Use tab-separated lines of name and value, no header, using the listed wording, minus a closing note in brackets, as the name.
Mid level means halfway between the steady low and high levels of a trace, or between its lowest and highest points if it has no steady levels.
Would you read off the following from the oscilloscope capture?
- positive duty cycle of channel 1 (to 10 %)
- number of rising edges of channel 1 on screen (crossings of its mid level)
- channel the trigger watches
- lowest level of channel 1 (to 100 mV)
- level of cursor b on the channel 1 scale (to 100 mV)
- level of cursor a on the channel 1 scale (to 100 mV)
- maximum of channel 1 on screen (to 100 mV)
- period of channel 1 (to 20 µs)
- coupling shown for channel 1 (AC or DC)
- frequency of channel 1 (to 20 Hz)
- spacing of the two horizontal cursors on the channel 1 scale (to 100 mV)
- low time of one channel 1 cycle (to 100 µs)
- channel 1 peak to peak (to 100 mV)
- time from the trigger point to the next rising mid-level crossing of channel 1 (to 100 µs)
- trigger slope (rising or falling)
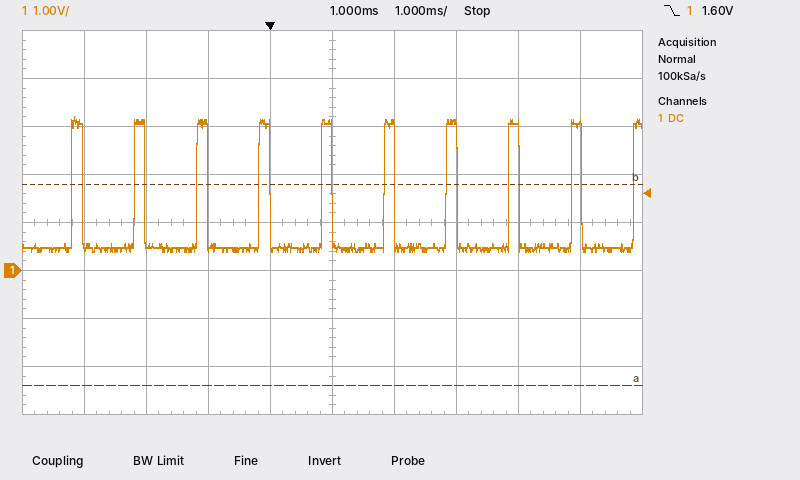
positive duty cycle of channel 1	20 %
number of rising edges of channel 1 on screen	10
channel the trigger watches	channel 1
lowest level of channel 1	400 mV
level of cursor b on the channel 1 scale	1.8 V
level of cursor a on the channel 1 scale	-2.4 V
maximum of channel 1 on screen	3.2 V
period of channel 1	1.00 ms
coupling shown for channel 1	DC
frequency of channel 1	1.00 kHz
spacing of the two horizontal cursors on the channel 1 scale	4.2 V
low time of one channel 1 cycle	800 µs
channel 1 peak to peak	2.8 V
time from the trigger point to the next rising mid-level crossing of channel 1	800 µs
trigger slope	falling
